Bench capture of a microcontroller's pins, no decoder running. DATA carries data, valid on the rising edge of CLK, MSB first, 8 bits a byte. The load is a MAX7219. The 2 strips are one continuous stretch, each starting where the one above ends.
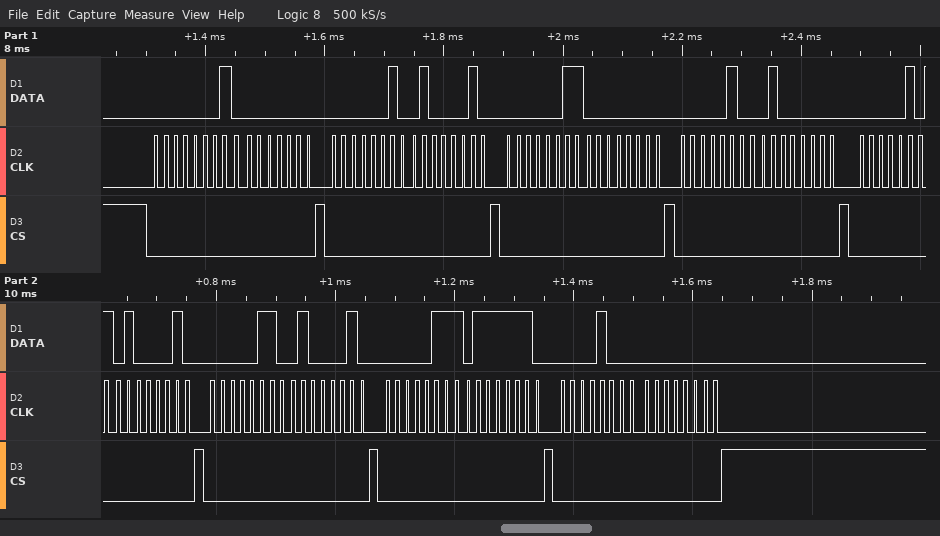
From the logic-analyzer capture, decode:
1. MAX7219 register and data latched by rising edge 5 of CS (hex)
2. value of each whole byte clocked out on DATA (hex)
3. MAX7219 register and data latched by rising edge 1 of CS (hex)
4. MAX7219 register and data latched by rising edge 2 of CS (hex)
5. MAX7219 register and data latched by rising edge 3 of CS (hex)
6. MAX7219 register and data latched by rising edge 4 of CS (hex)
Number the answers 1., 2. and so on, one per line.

1. register 0x5, data 0x42
2. 01 00 02 42 03 00 04 40 05 42 06 42 07 7E 08 00
3. register 0x1, data 0x00
4. register 0x2, data 0x42
5. register 0x3, data 0x00
6. register 0x4, data 0x40
